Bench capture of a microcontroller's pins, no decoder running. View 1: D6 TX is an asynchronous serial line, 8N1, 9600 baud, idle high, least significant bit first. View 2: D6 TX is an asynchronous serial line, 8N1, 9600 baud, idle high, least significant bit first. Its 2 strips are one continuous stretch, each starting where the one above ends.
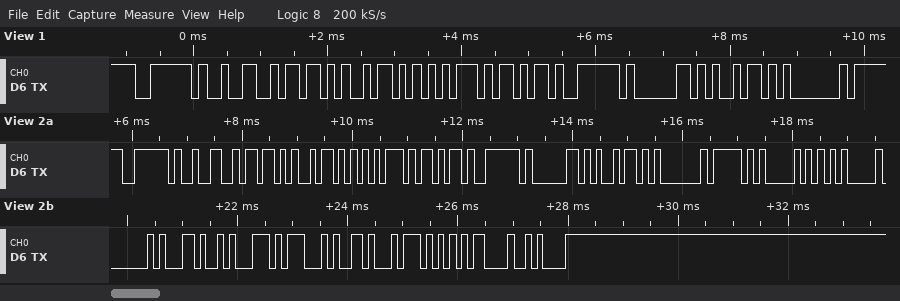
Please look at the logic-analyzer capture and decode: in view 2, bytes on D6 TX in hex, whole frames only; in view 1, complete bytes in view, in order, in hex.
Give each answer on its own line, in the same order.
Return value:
7E 32 5B 5A 75 6B 7E 60 69 01 5F 50 05 40 2C 71 47 16 57 0D 0A
7E 32 5B 5A 75 6B 7E 60 69 01
